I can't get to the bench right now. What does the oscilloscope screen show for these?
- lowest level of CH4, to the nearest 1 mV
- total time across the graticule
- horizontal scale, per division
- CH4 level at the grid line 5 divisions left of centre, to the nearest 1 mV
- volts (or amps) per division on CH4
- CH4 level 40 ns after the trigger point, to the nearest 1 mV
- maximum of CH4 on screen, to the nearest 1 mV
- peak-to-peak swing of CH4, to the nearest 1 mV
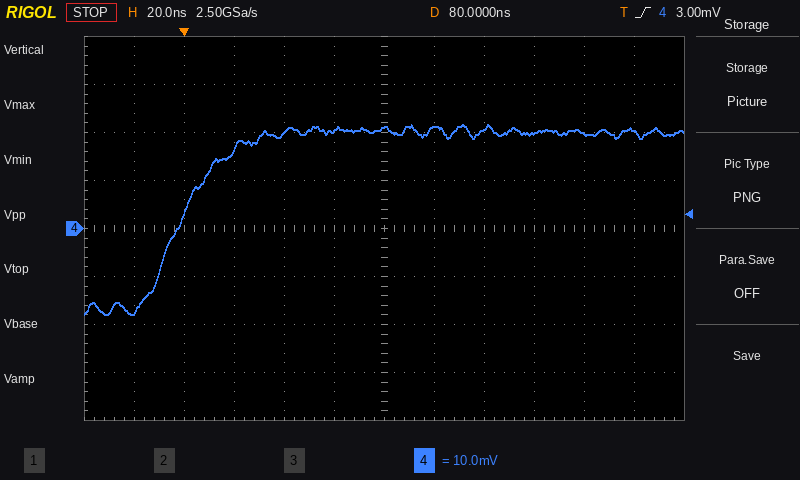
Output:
-18 mV
240 ns
20 ns
-17 mV
10 mV
20 mV
22 mV
40 mV
